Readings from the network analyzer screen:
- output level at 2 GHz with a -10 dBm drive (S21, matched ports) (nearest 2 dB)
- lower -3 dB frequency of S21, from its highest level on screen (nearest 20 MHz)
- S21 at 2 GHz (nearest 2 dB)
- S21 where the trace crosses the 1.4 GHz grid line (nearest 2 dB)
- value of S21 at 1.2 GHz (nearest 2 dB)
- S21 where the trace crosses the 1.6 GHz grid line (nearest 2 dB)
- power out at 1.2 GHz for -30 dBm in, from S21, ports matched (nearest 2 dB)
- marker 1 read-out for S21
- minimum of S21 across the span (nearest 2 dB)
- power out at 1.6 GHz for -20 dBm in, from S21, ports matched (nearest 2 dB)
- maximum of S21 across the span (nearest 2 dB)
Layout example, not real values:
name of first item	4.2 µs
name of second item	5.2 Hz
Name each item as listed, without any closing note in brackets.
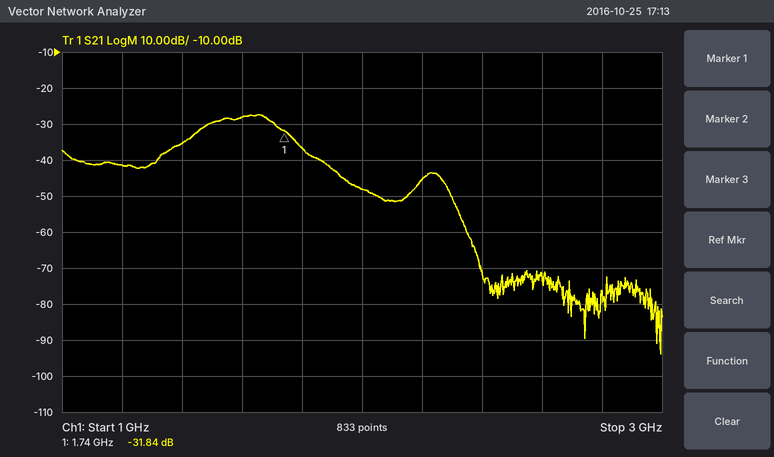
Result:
output level at 2 GHz with a -10 dBm drive (S21, matched ports)	-58 dBm
lower -3 dB frequency of S21, from its highest level on screen	1.48 GHz
S21 at 2 GHz	-48 dB
S21 where the trace crosses the 1.4 GHz grid line	-36 dB
value of S21 at 1.2 GHz	-42 dB
S21 where the trace crosses the 1.6 GHz grid line	-28 dB
power out at 1.2 GHz for -30 dBm in, from S21, ports matched	-72 dBm
marker 1 read-out for S21	-31.84 dB
minimum of S21 across the span	-94 dB
power out at 1.6 GHz for -20 dBm in, from S21, ports matched	-48 dBm
maximum of S21 across the span	-28 dB
